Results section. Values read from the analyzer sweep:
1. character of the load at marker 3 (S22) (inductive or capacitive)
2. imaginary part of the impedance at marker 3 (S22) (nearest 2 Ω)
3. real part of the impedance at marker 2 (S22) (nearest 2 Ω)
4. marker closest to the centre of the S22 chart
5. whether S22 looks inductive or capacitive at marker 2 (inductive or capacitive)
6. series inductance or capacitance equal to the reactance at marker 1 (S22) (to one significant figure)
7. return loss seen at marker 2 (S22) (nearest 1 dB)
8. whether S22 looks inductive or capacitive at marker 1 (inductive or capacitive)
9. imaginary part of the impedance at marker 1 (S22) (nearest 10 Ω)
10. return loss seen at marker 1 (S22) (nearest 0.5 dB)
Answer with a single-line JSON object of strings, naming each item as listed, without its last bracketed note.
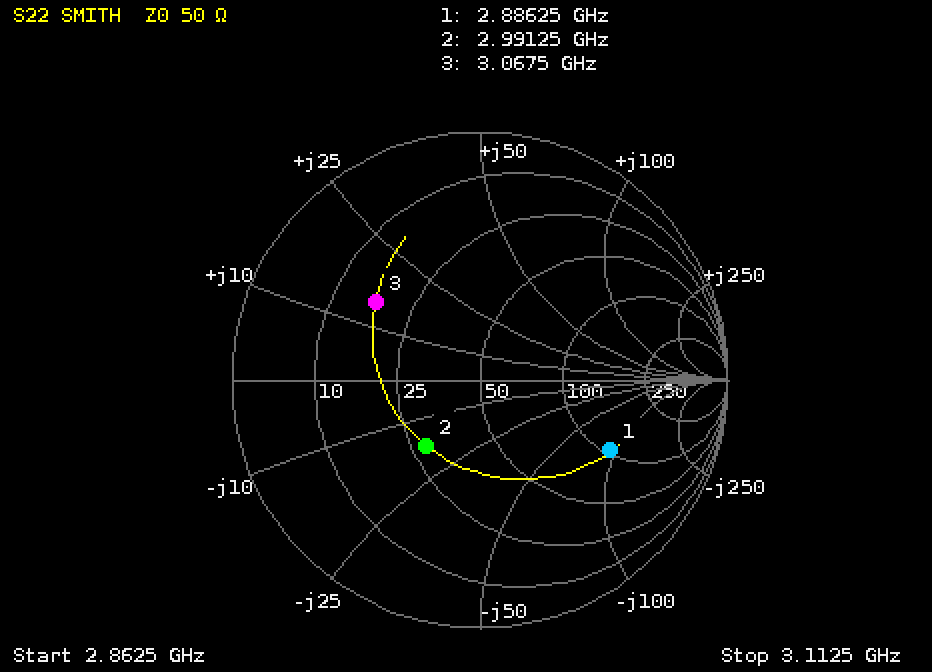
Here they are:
{"character of the load at marker 3 (S22)": "inductive", "imaginary part of the impedance at marker 3 (S22)": "+14 Ω", "real part of the impedance at marker 2 (S22)": "28 Ω", "marker closest to the centre of the S22 chart": "marker 2", "whether S22 looks inductive or capacitive at marker 2": "capacitive", "series inductance or capacitance equal to the reactance at marker 1 (S22)": "600 fF", "return loss seen at marker 2 (S22)": "9 dB", "whether S22 looks inductive or capacitive at marker 1": "capacitive", "imaginary part of the impedance at marker 1 (S22)": "-90 Ω", "return loss seen at marker 1 (S22)": "4.5 dB"}
